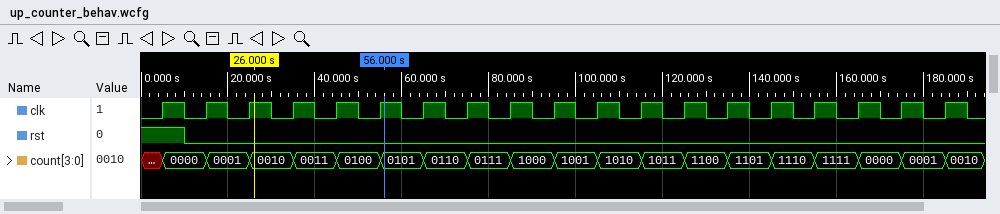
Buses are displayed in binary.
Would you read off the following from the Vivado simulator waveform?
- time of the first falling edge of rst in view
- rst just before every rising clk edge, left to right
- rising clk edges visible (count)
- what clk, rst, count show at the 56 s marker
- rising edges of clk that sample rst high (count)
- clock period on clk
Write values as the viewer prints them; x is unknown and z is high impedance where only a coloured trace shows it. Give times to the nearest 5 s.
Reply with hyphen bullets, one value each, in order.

- 10 s
- 1 0 0 0 0 0 0 0 0 0 0 0 0 0 0 0 0 0 0
- 19
- clk=1, rst=0, count=0101
- 1
- 10 s
